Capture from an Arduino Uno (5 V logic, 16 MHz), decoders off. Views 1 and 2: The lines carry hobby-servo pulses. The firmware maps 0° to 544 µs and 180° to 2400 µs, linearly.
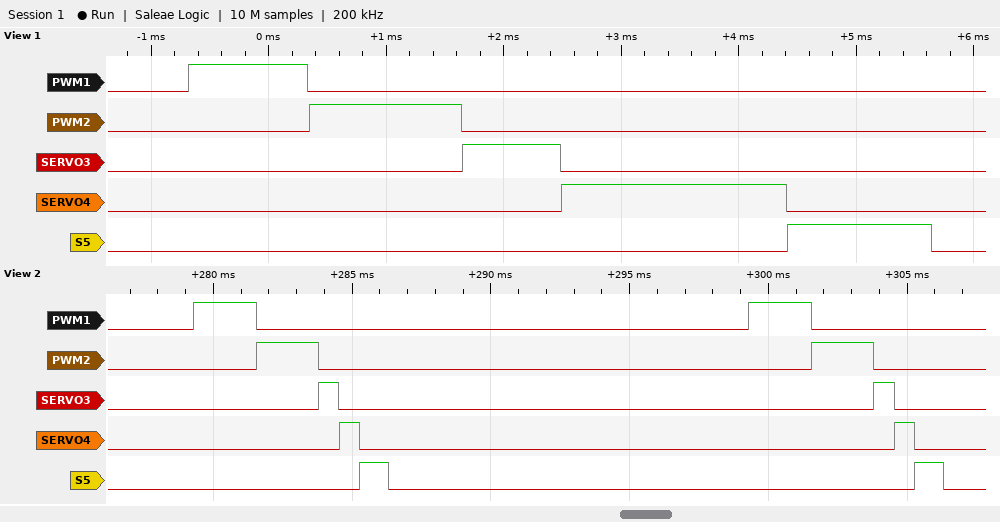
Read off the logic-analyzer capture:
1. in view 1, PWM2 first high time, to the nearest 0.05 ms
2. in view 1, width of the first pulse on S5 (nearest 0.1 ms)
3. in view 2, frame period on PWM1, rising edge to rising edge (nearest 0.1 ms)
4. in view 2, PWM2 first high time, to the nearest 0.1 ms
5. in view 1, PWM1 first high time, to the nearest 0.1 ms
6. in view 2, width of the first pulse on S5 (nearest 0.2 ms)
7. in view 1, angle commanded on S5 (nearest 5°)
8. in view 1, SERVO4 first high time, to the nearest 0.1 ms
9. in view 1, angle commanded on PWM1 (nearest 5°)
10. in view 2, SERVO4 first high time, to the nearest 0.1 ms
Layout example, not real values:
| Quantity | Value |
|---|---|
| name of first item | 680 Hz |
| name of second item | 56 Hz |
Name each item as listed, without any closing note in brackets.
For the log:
| Quantity | Value |
|---|---|
| in view 1, PWM2 first high time, to the nearest 0.05 ms | 1.30 ms |
| in view 1, width of the first pulse on S5 | 1.2 ms |
| in view 2, frame period on PWM1, rising edge to rising edge | 20.0 ms |
| in view 2, PWM2 first high time, to the nearest 0.1 ms | 2.2 ms |
| in view 1, PWM1 first high time, to the nearest 0.1 ms | 1.0 ms |
| in view 2, width of the first pulse on S5 | 1.0 ms |
| in view 1, angle commanded on S5 | 65° |
| in view 1, SERVO4 first high time, to the nearest 0.1 ms | 1.9 ms |
| in view 1, angle commanded on PWM1 | 45° |
| in view 2, SERVO4 first high time, to the nearest 0.1 ms | 0.7 ms |
